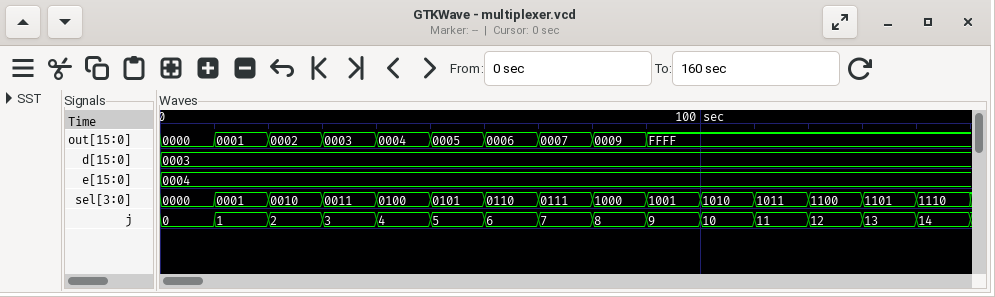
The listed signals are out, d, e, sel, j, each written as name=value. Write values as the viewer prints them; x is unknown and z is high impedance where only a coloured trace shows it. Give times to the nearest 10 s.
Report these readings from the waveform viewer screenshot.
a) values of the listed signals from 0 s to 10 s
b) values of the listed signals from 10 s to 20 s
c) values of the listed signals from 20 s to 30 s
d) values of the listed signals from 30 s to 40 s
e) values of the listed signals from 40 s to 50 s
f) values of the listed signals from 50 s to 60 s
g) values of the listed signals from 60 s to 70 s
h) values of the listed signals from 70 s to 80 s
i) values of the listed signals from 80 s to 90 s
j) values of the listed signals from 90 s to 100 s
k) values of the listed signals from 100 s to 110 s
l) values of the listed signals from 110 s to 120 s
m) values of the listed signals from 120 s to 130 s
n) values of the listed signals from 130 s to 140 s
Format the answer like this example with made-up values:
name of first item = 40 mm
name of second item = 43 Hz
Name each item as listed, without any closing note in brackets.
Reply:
values of the listed signals from 0 s to 10 s = out=0000, d=0003, e=0004, sel=0000, j=0
values of the listed signals from 10 s to 20 s = out=0001, d=0003, e=0004, sel=0001, j=1
values of the listed signals from 20 s to 30 s = out=0002, d=0003, e=0004, sel=0010, j=2
values of the listed signals from 30 s to 40 s = out=0003, d=0003, e=0004, sel=0011, j=3
values of the listed signals from 40 s to 50 s = out=0004, d=0003, e=0004, sel=0100, j=4
values of the listed signals from 50 s to 60 s = out=0005, d=0003, e=0004, sel=0101, j=5
values of the listed signals from 60 s to 70 s = out=0006, d=0003, e=0004, sel=0110, j=6
values of the listed signals from 70 s to 80 s = out=0007, d=0003, e=0004, sel=0111, j=7
values of the listed signals from 80 s to 90 s = out=0009, d=0003, e=0004, sel=1000, j=8
values of the listed signals from 90 s to 100 s = out=FFFF, d=0003, e=0004, sel=1001, j=9
values of the listed signals from 100 s to 110 s = out=FFFF, d=0003, e=0004, sel=1010, j=10
values of the listed signals from 110 s to 120 s = out=FFFF, d=0003, e=0004, sel=1011, j=11
values of the listed signals from 120 s to 130 s = out=FFFF, d=0003, e=0004, sel=1100, j=12
values of the listed signals from 130 s to 140 s = out=FFFF, d=0003, e=0004, sel=1101, j=13
